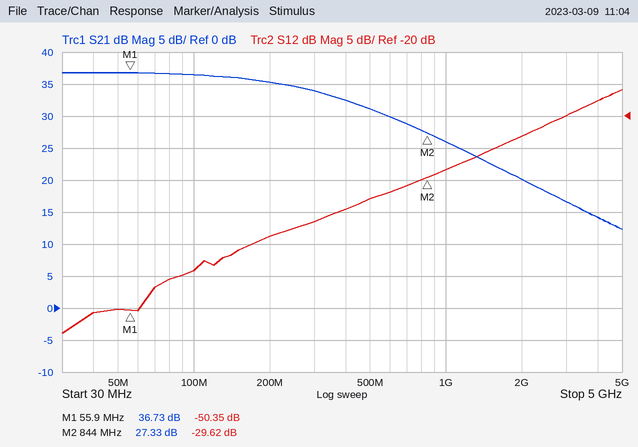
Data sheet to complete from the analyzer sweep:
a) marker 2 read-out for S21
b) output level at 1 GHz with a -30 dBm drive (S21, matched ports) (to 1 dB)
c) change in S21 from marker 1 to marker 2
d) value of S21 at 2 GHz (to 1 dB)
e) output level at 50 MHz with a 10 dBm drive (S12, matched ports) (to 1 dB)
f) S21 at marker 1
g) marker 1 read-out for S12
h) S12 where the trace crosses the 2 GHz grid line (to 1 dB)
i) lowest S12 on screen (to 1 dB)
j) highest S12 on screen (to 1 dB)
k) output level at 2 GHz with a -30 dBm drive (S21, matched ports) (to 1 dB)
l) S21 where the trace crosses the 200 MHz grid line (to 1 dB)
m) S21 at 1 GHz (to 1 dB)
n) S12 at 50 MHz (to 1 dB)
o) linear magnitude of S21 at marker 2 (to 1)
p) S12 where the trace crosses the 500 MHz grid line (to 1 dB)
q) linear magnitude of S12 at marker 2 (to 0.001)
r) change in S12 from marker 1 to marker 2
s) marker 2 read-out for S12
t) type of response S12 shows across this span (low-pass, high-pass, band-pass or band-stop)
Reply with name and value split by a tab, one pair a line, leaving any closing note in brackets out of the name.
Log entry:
marker 2 read-out for S21	27.33 dB
output level at 1 GHz with a -30 dBm drive (S21, matched ports)	-4 dBm
change in S21 from marker 1 to marker 2	-9.40 dB
value of S21 at 2 GHz	20 dB
output level at 50 MHz with a 10 dBm drive (S12, matched ports)	-40 dBm
S21 at marker 1	36.73 dB
marker 1 read-out for S12	-50.35 dB
S12 where the trace crosses the 2 GHz grid line	-23 dB
lowest S12 on screen	-54 dB
highest S12 on screen	-16 dB
output level at 2 GHz with a -30 dBm drive (S21, matched ports)	-10 dBm
S21 where the trace crosses the 200 MHz grid line	35 dB
S21 at 1 GHz	26 dB
S12 at 50 MHz	-50 dB
linear magnitude of S21 at marker 2	23
S12 where the trace crosses the 500 MHz grid line	-33 dB
linear magnitude of S12 at marker 2	0.033
change in S12 from marker 1 to marker 2	20.73 dB
marker 2 read-out for S12	-29.62 dB
type of response S12 shows across this span	high-pass
